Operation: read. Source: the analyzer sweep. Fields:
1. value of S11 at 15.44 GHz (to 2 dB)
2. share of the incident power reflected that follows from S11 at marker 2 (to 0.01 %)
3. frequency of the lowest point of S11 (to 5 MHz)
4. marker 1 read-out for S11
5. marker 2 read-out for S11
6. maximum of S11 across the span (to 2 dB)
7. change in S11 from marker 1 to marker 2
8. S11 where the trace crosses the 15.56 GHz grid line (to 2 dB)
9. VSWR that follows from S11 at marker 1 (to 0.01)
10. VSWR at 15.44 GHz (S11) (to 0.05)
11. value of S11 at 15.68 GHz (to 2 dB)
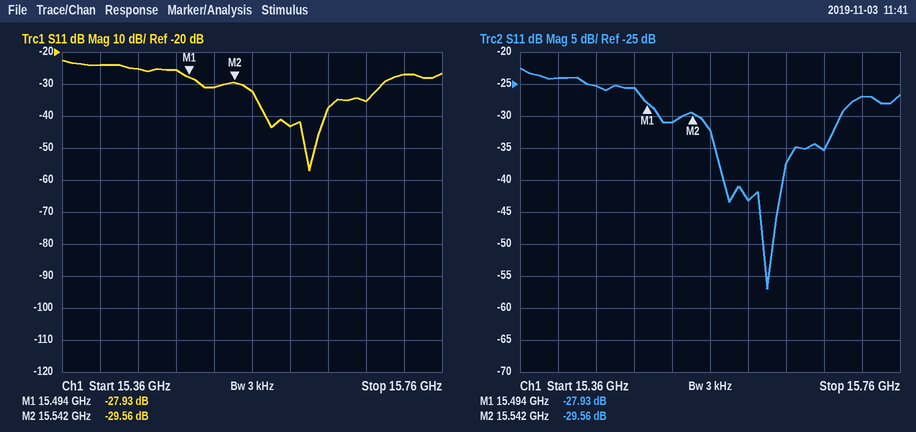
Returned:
-26 dB
0.11 %
15.620 GHz
-27.93 dB
-29.56 dB
-22 dB
-1.63 dB
-32 dB
1.08
1.10
-36 dB
